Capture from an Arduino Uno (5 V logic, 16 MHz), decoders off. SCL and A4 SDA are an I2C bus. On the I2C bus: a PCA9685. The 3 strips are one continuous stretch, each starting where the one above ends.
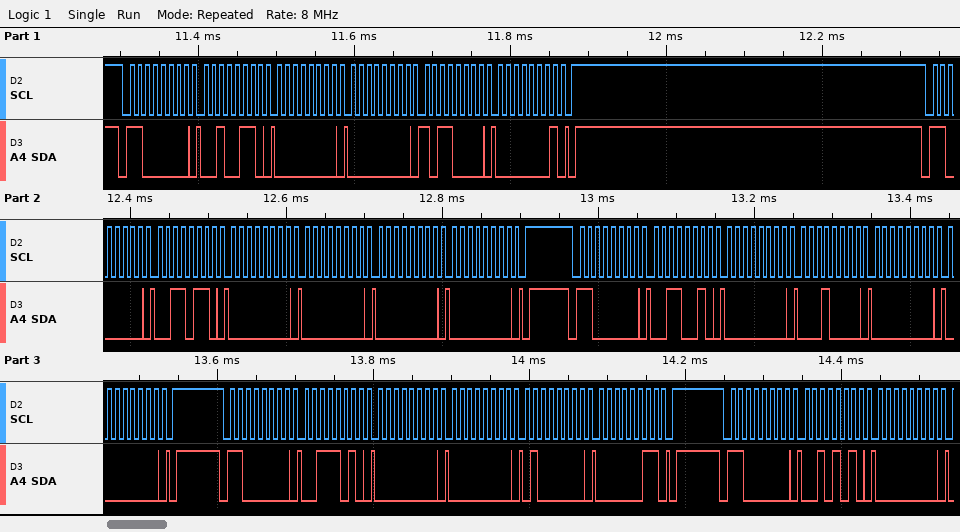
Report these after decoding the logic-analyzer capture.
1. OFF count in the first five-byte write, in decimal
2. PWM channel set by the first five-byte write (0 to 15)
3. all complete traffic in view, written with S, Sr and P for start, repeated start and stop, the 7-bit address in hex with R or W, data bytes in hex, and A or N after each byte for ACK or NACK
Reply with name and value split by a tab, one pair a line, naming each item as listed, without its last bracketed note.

OFF count in the first five-byte write, in decimal	432
PWM channel set by the first five-byte write	8
all complete traffic in view, written with S, Sr and P for start, repeated start and stop, the 7-bit address in hex with R or W, data bytes in hex, and A or N after each byte for ACK or NACK	S 60W A 26 A 00 A 00 A B0 A 01 A P S 60W A 36 A 00 A 00 A 00 A 00 A P S 60W A 32 A 00 A 10 A 00 A 00 A P S 60W A 3A A 00 A 00 A 40 A 03 A P S 60W A 2A A 00 A
